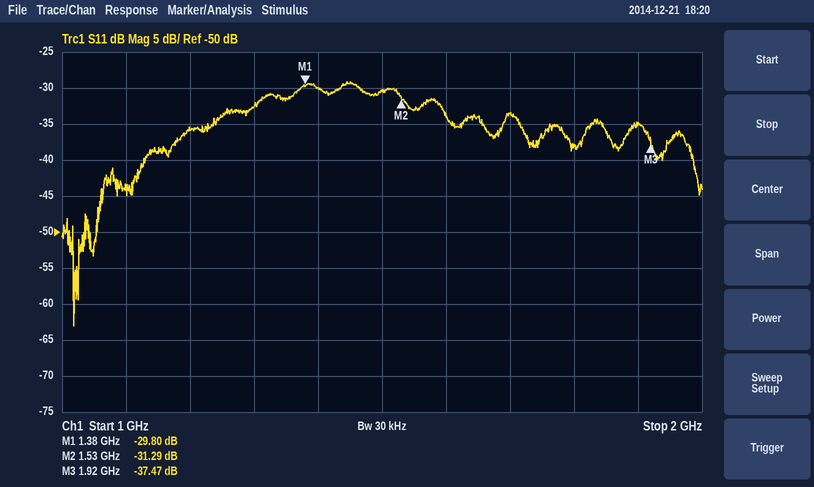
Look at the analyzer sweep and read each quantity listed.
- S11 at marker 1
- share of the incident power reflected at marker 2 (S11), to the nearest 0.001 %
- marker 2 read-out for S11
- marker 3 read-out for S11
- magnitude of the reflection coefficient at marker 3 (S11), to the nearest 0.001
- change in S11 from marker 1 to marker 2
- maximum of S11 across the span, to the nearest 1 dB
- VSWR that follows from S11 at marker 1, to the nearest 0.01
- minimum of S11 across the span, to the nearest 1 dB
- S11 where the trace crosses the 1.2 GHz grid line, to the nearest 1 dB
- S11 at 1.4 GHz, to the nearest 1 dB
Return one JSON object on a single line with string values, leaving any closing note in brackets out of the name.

{"S11 at marker 1": "-29.80 dB", "share of the incident power reflected at marker 2 (S11), to the nearest 0.001 %": "0.074 %", "marker 2 read-out for S11": "-31.29 dB", "marker 3 read-out for S11": "-37.47 dB", "magnitude of the reflection coefficient at marker 3 (S11), to the nearest 0.001": "0.013", "change in S11 from marker 1 to marker 2": "-1.49 dB", "maximum of S11 across the span, to the nearest 1 dB": "-29 dB", "VSWR that follows from S11 at marker 1, to the nearest 0.01": "1.07", "minimum of S11 across the span, to the nearest 1 dB": "-63 dB", "S11 where the trace crosses the 1.2 GHz grid line, to the nearest 1 dB": "-36 dB", "S11 at 1.4 GHz, to the nearest 1 dB": "-30 dB"}
